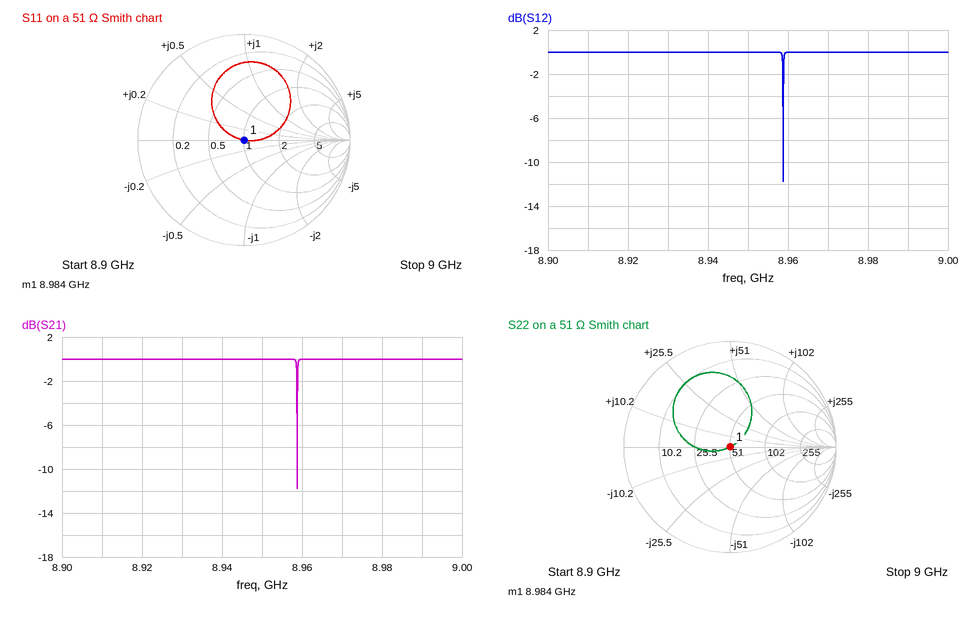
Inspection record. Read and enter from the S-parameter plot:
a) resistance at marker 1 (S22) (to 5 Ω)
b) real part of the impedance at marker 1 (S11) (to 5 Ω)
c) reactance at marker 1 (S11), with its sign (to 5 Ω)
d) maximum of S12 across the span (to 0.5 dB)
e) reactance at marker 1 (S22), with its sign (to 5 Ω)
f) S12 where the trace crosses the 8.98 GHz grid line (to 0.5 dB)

50 Ω
50 Ω
0 Ω
0.0 dB
0 Ω
0.0 dB
